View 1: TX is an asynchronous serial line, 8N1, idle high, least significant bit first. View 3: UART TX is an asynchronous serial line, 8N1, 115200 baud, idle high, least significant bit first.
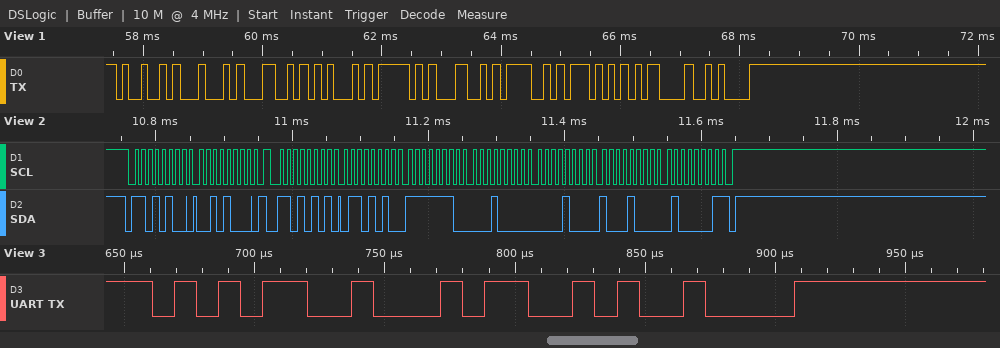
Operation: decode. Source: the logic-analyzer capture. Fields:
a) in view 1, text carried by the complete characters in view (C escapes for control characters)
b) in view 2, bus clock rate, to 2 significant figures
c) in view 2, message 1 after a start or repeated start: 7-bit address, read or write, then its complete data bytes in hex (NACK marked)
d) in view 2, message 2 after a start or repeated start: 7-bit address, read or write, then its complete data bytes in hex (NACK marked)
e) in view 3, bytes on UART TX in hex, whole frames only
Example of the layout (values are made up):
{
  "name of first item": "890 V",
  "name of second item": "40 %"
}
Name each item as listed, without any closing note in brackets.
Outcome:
{
  "in view 1, text carried by the complete characters in view": "\"IDLE_LOW\\r\\n\"",
  "in view 2, bus clock rate, to 2 significant figures": "100 kHz",
  "in view 2, message 1 after a start or repeated start: 7-bit address, read or write, then its complete data bytes in hex": "0x6A write: 28",
  "in view 2, message 2 after a start or repeated start: 7-bit address, read or write, then its complete data bytes in hex": "0x6A read: 6A FE 10 08 88 41 NACK",
  "in view 3, bytes on UART TX in hex, whole frames only": "35 34 09"
}
